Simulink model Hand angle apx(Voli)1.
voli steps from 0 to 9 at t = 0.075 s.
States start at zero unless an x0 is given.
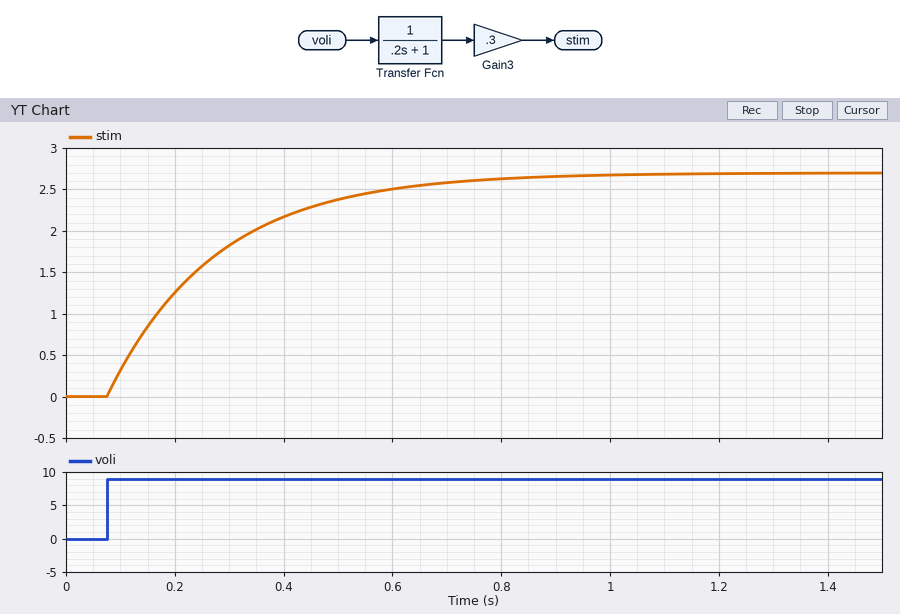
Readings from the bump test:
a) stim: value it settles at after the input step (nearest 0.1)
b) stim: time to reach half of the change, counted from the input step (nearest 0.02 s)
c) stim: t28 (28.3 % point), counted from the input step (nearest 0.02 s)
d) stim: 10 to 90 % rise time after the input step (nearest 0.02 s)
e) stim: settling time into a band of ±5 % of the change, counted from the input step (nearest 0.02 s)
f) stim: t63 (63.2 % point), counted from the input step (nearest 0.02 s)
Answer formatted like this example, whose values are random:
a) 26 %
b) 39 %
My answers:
a) 2.7
b) 0.14 s
c) 0.06 s
d) 0.44 s
e) 0.60 s
f) 0.20 s
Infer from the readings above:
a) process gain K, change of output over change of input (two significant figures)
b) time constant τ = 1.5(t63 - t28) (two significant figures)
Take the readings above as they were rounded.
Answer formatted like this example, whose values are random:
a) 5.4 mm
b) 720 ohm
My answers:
a) 0.30
b) 0.21 s
